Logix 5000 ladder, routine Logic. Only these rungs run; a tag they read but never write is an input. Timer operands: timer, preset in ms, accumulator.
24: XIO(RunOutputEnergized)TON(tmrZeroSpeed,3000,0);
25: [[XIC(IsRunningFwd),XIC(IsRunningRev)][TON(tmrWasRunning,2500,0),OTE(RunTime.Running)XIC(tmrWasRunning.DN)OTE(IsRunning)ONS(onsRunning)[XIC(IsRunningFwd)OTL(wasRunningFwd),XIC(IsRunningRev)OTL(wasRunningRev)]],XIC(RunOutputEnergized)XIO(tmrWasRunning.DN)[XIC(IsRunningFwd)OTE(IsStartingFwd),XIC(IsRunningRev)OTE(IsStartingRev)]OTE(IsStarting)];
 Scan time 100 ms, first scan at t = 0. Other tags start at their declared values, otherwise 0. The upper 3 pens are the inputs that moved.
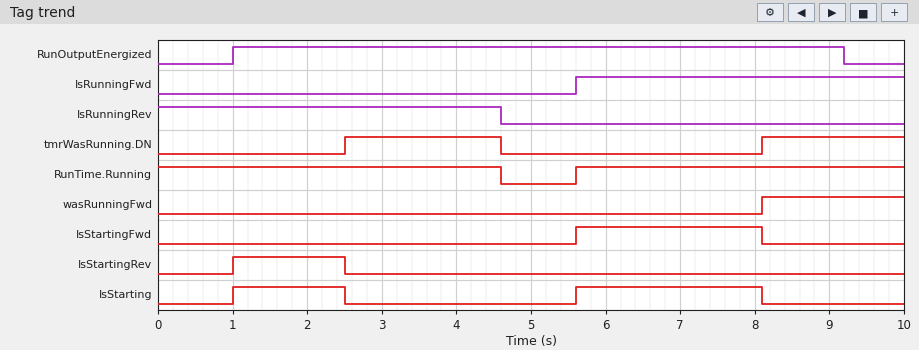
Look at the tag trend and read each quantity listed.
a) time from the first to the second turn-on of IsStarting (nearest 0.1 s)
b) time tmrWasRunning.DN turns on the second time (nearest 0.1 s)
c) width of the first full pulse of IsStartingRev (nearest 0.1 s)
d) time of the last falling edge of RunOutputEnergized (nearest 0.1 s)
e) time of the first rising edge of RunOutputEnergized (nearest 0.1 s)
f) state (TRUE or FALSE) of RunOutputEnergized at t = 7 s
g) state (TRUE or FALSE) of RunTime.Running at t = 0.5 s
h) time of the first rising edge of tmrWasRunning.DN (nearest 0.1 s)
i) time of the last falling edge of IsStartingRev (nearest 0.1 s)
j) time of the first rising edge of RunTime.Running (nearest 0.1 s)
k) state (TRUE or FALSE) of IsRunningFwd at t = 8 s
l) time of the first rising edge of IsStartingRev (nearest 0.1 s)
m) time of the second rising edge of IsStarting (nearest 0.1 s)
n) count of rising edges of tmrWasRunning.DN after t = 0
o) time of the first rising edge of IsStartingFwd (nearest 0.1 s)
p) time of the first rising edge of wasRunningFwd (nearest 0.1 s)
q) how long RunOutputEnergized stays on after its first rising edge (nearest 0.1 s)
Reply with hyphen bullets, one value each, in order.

- 4.6 s
- 8.1 s
- 1.5 s
- 9.2 s
- 1.0 s
- TRUE
- TRUE
- 2.5 s
- 2.5 s
- 5.6 s
- TRUE
- 1.0 s
- 5.6 s
- 2
- 5.6 s
- 8.1 s
- 8.2 s
